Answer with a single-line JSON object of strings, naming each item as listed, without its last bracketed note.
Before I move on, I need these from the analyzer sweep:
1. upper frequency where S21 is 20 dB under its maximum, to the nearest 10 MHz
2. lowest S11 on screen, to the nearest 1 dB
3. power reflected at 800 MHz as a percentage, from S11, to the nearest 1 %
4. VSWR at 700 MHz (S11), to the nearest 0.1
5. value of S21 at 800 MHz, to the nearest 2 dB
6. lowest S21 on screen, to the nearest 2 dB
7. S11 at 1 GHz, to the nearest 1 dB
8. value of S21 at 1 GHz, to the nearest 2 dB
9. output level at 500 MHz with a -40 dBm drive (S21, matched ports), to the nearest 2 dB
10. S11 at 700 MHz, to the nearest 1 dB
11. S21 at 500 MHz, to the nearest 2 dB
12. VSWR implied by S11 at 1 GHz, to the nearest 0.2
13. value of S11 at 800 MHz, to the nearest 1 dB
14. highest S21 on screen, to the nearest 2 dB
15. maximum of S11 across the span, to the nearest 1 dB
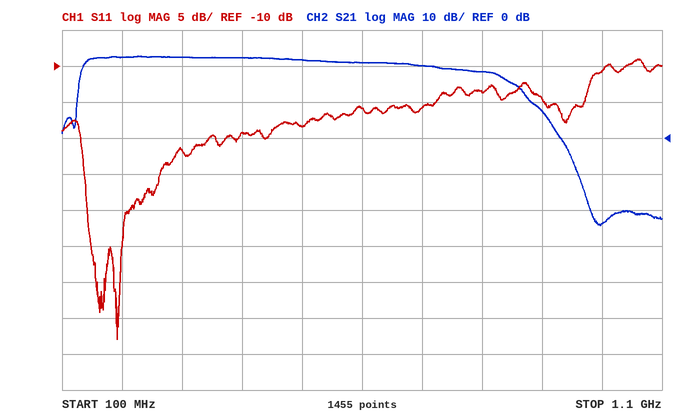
{"upper frequency where S21 is 20 dB under its maximum, to the nearest 10 MHz": "920 MHz", "lowest S11 on screen, to the nearest 1 dB": "-48 dB", "power reflected at 800 MHz as a percentage, from S11, to the nearest 1 %": "4 %", "VSWR at 700 MHz (S11), to the nearest 0.1": "1.4", "value of S21 at 800 MHz, to the nearest 2 dB": "18 dB", "lowest S21 on screen, to the nearest 2 dB": "-24 dB", "S11 at 1 GHz, to the nearest 1 dB": "-11 dB", "value of S21 at 1 GHz, to the nearest 2 dB": "-24 dB", "output level at 500 MHz with a -40 dBm drive (S21, matched ports), to the nearest 2 dB": "-18 dBm", "S11 at 700 MHz, to the nearest 1 dB": "-16 dB", "S21 at 500 MHz, to the nearest 2 dB": "22 dB", "VSWR implied by S11 at 1 GHz, to the nearest 0.2": "1.8", "value of S11 at 800 MHz, to the nearest 1 dB": "-14 dB", "highest S21 on screen, to the nearest 2 dB": "22 dB", "maximum of S11 across the span, to the nearest 1 dB": "-9 dB"}
